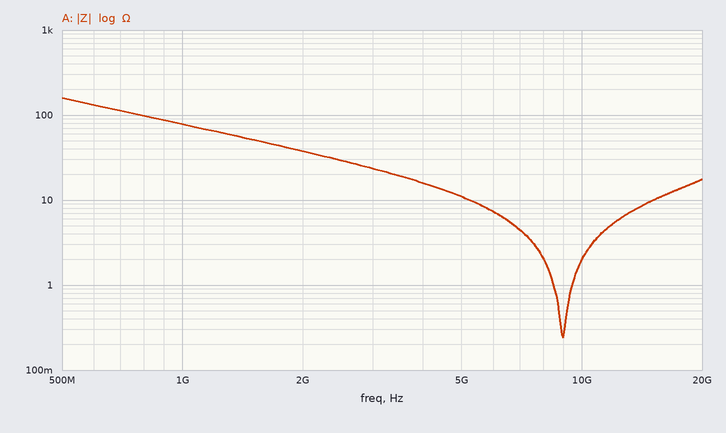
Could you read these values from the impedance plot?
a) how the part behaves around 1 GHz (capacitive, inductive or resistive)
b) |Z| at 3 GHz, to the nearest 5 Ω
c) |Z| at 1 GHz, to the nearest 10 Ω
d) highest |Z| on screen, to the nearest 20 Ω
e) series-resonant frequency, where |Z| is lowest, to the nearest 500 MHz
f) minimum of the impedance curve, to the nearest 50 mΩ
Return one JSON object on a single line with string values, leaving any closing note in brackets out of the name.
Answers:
{"how the part behaves around 1 GHz": "capacitive", "|Z| at 3 GHz, to the nearest 5 Ω": "25 Ω", "|Z| at 1 GHz, to the nearest 10 Ω": "80 Ω", "highest |Z| on screen, to the nearest 20 Ω": "160 Ω", "series-resonant frequency, where |Z| is lowest, to the nearest 500 MHz": "9.0 GHz", "minimum of the impedance curve, to the nearest 50 mΩ": "250 mΩ"}
